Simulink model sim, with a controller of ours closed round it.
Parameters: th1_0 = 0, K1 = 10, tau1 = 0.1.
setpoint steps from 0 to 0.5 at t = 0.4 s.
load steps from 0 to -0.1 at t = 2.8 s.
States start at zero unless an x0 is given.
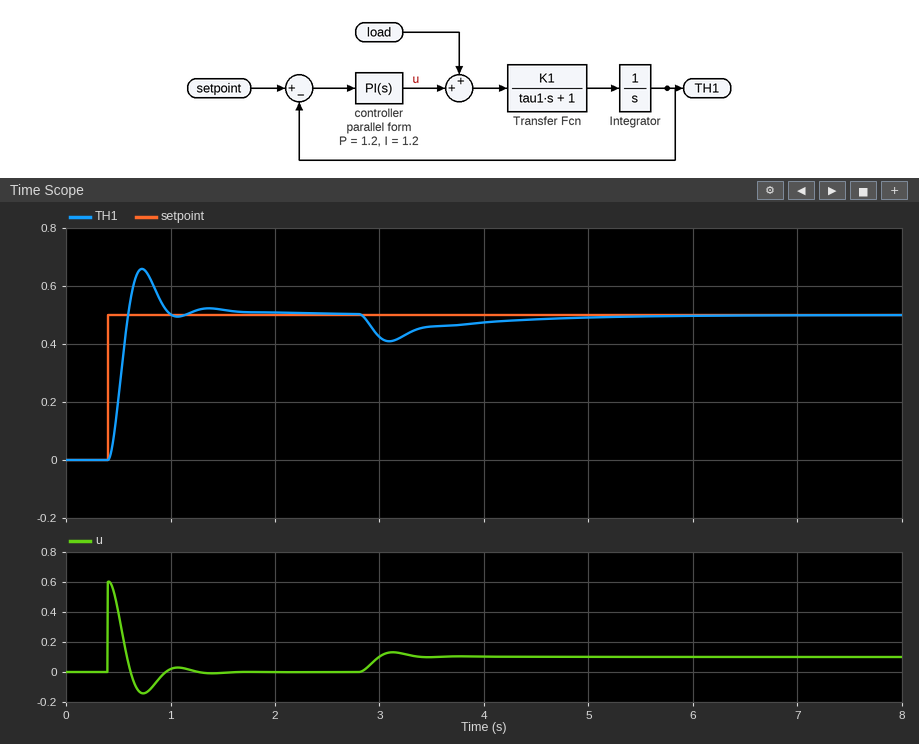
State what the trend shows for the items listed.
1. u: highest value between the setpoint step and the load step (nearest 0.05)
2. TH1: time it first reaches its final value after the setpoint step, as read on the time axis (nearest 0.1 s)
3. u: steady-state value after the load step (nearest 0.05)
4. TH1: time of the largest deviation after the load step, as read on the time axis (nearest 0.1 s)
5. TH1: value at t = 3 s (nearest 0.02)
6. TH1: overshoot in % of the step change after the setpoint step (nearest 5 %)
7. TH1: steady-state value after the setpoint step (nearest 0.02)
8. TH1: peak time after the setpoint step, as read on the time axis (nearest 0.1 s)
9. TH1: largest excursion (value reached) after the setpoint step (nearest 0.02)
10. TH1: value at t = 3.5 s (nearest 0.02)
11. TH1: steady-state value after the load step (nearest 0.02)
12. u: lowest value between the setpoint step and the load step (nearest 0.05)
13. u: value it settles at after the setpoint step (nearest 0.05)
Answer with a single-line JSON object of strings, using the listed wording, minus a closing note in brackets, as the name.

{"u: highest value between the setpoint step and the load step": "0.60", "TH1: time it first reaches its final value after the setpoint step, as read on the time axis": "0.6 s", "u: steady-state value after the load step": "0.10", "TH1: time of the largest deviation after the load step, as read on the time axis": "3.1 s", "TH1: value at t = 3 s": "0.42", "TH1: overshoot in % of the step change after the setpoint step": "30 %", "TH1: steady-state value after the setpoint step": "0.50", "TH1: peak time after the setpoint step, as read on the time axis": "0.7 s", "TH1: largest excursion (value reached) after the setpoint step": "0.66", "TH1: value at t = 3.5 s": "0.46", "TH1: steady-state value after the load step": "0.50", "u: lowest value between the setpoint step and the load step": "-0.15", "u: value it settles at after the setpoint step": "0.00"}
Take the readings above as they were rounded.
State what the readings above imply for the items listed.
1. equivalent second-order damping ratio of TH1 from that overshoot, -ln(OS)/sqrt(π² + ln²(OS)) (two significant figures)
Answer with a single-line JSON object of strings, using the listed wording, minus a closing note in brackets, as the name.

{"equivalent second-order damping ratio of TH1 from that overshoot, -ln(OS)/sqrt(π² + ln²(OS))": "0.36"}
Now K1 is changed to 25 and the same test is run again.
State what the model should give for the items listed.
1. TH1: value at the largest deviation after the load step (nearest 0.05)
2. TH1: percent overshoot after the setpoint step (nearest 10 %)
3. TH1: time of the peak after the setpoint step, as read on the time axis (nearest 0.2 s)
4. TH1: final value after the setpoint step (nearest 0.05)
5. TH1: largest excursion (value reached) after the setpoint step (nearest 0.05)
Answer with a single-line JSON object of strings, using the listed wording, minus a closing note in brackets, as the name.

{"TH1: value at the largest deviation after the load step": "0.40", "TH1: percent overshoot after the setpoint step": "50 %", "TH1: time of the peak after the setpoint step, as read on the time axis": "0.6 s", "TH1: final value after the setpoint step": "0.50", "TH1: largest excursion (value reached) after the setpoint step": "0.75"}
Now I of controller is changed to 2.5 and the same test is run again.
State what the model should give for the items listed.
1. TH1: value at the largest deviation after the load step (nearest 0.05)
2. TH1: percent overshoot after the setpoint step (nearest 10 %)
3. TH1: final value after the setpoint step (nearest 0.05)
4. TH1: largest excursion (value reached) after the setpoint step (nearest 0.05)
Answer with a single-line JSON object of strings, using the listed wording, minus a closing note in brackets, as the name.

{"TH1: value at the largest deviation after the load step": "0.40", "TH1: percent overshoot after the setpoint step": "40 %", "TH1: final value after the setpoint step": "0.50", "TH1: largest excursion (value reached) after the setpoint step": "0.70"}
